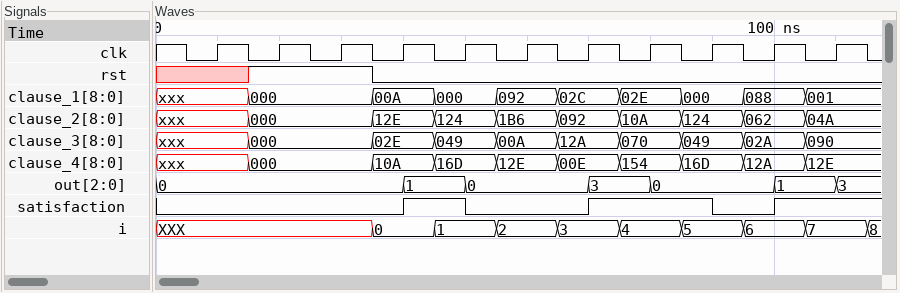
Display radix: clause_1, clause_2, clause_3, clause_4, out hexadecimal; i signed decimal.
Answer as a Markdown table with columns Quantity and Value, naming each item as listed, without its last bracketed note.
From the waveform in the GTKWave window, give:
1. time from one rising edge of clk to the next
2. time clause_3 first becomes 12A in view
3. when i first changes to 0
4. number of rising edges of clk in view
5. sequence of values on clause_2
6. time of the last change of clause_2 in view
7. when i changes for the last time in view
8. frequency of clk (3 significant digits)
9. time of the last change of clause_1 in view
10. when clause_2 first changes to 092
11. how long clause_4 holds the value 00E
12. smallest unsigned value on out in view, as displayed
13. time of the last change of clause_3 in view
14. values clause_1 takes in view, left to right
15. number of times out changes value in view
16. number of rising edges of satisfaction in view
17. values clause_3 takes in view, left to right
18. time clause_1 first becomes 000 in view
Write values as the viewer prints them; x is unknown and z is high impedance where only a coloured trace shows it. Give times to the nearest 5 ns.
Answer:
| Quantity | Value |
|---|---|
| time from one rising edge of clk to the next | 10 ns |
| time clause_3 first becomes 12A in view | 65 ns |
| when i first changes to 0 | 35 ns |
| number of rising edges of clk in view | 11 |
| sequence of values on clause_2 | xxx, 000, 12E, 124, 1B6, 092, 10A, 124, 062, 04A |
| time of the last change of clause_2 in view | 105 ns |
| when i changes for the last time in view | 115 ns |
| frequency of clk | 100 MHz |
| time of the last change of clause_1 in view | 105 ns |
| when clause_2 first changes to 092 | 65 ns |
| how long clause_4 holds the value 00E | 10 ns |
| smallest unsigned value on out in view, as displayed | 0 |
| time of the last change of clause_3 in view | 105 ns |
| values clause_1 takes in view, left to right | xxx, 000, 00A, 000, 092, 02C, 02E, 000, 088, 001 |
| number of times out changes value in view | 6 |
| number of rising edges of satisfaction in view | 3 |
| values clause_3 takes in view, left to right | xxx, 000, 02E, 049, 00A, 12A, 070, 049, 02A, 090 |
| time clause_1 first becomes 000 in view | 15 ns |
